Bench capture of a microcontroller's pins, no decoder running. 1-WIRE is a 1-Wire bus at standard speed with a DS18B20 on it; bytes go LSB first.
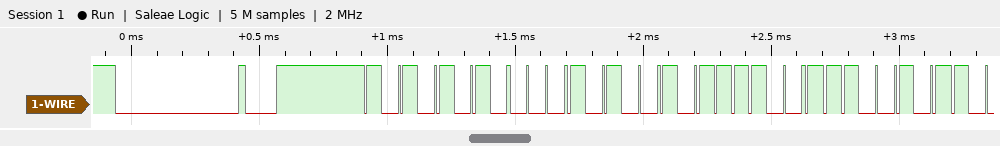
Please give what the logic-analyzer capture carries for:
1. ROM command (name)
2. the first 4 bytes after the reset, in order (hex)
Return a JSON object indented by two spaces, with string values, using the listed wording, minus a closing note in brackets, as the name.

{
  "ROM command": "Match ROM",
  "the first 4 bytes after the reset, in order": "55 28 3D A7"
}
